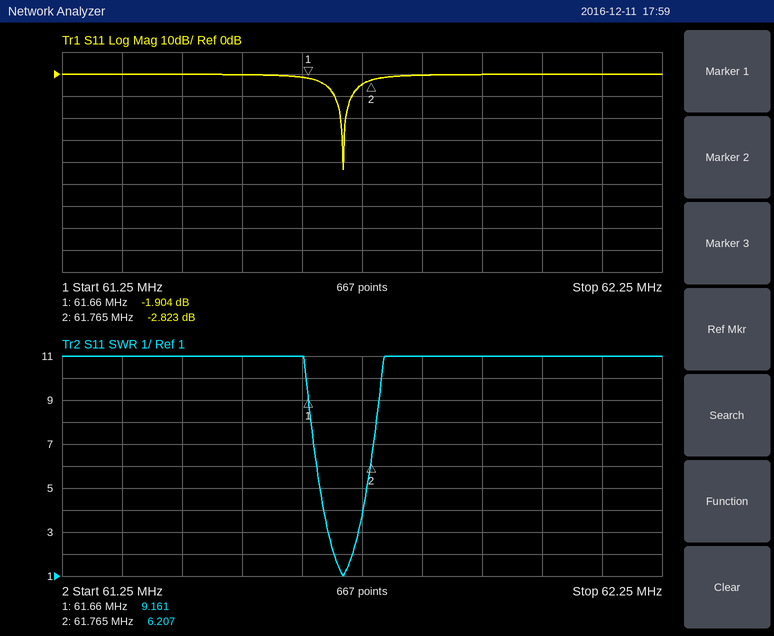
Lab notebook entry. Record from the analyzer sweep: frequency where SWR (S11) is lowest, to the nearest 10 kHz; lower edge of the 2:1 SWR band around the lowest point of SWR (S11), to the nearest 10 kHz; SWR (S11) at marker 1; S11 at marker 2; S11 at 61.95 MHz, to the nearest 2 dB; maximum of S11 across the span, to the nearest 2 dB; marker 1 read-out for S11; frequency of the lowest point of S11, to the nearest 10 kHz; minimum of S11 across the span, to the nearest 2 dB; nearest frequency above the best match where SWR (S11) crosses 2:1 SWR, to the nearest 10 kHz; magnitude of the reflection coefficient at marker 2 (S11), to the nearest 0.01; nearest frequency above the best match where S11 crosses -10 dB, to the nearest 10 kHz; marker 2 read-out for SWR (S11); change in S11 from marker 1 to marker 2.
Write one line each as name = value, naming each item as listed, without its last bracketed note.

frequency where SWR (S11) is lowest, to the nearest 10 kHz = 61.72 MHz
lower edge of the 2:1 SWR band around the lowest point of SWR (S11), to the nearest 10 kHz = 61.70 MHz
SWR (S11) at marker 1 = 9.161
S11 at marker 2 = -2.823 dB
S11 at 61.95 MHz, to the nearest 2 dB = 0 dB
maximum of S11 across the span, to the nearest 2 dB = 0 dB
marker 1 read-out for S11 = -1.904 dB
frequency of the lowest point of S11, to the nearest 10 kHz = 61.72 MHz
minimum of S11 across the span, to the nearest 2 dB = -44 dB
nearest frequency above the best match where SWR (S11) crosses 2:1 SWR, to the nearest 10 kHz = 61.73 MHz
magnitude of the reflection coefficient at marker 2 (S11), to the nearest 0.01 = 0.72
nearest frequency above the best match where S11 crosses -10 dB, to the nearest 10 kHz = 61.73 MHz
marker 2 read-out for SWR = 6.207
change in S11 from marker 1 to marker 2 = -0.919 dB
